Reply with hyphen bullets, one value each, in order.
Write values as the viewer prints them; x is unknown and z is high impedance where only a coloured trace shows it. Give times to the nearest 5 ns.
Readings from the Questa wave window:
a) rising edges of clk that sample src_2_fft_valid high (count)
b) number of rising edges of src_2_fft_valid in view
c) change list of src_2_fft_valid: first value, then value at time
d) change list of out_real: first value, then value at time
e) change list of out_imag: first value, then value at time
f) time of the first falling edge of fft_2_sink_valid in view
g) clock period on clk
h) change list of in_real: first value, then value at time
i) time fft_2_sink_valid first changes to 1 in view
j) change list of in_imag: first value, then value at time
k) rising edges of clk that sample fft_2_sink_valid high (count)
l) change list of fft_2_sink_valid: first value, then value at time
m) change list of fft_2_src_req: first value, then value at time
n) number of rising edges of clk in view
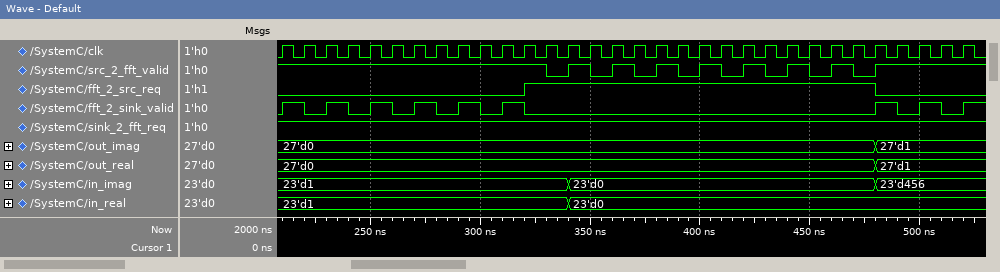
- 24
- 8
- 1, 0 at 330 ns, 1 at 340 ns, 0 at 350 ns, 1 at 360 ns, 0 at 370 ns, 1 at 380 ns, 0 at 390 ns, 1 at 400 ns, 0 at 410 ns, 1 at 420 ns, 0 at 430 ns, 1 at 440 ns, 0 at 450 ns, 1 at 460 ns, 0 at 470 ns, 1 at 480 ns
- 27'd0, 27'd1 at 480 ns
- 27'd0, 27'd1 at 480 ns
- 220 ns
- 10 ns
- 23'd1, 23'd0 at 340 ns
- 210 ns
- 23'd1, 23'd0 at 340 ns, 23'd456 at 480 ns
- 8
- 0, 1 at 210 ns, 0 at 220 ns, 1 at 230 ns, 0 at 240 ns, 1 at 250 ns, 0 at 260 ns, 1 at 270 ns, 0 at 280 ns, 1 at 290 ns, 0 at 300 ns, 1 at 310 ns, 0 at 320 ns, 1 at 480 ns, 0 at 490 ns, 1 at 500 ns, 0 at 510 ns, 1 at 520 ns
- 0, 1 at 320 ns, 0 at 480 ns
- 32
